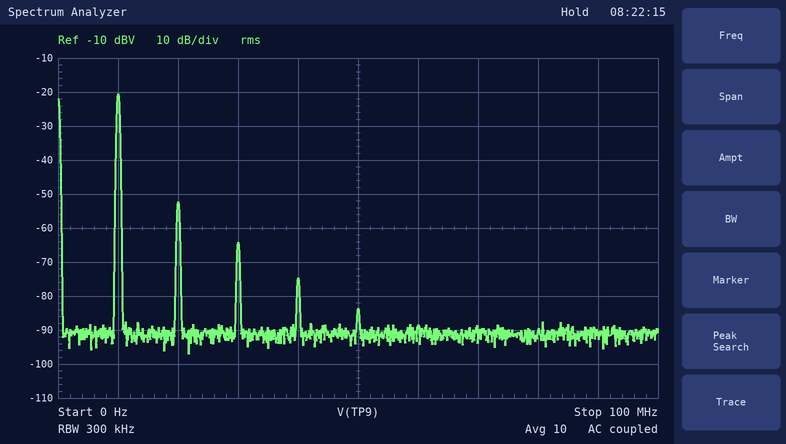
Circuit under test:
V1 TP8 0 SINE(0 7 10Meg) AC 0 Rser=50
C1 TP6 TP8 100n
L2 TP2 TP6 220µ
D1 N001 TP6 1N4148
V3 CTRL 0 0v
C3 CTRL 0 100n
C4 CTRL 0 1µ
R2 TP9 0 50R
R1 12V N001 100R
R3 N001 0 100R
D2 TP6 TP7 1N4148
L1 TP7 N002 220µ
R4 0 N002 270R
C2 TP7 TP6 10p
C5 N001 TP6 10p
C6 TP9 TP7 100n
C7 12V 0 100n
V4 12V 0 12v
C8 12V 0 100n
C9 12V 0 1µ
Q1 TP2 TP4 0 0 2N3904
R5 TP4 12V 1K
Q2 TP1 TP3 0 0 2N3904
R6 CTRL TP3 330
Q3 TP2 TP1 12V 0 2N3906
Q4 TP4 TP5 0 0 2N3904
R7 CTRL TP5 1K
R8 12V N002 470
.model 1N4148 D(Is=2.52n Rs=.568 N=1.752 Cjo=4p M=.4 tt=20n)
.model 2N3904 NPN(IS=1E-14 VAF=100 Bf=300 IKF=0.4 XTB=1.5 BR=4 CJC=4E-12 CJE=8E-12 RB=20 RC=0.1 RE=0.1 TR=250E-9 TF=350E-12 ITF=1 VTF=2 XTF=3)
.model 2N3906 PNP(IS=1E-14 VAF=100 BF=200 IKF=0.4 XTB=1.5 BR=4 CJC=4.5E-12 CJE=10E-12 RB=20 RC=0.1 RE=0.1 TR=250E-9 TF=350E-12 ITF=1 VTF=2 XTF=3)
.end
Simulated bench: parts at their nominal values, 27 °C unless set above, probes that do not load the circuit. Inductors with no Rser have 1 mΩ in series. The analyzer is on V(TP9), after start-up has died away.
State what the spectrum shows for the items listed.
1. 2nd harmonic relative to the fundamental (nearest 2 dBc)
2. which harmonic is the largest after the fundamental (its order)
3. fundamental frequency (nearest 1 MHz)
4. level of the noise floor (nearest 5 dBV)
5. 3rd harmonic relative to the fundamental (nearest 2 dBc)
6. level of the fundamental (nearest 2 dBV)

-32 dBc
2
10 MHz
-90 dBV
-44 dBc
-20 dBV
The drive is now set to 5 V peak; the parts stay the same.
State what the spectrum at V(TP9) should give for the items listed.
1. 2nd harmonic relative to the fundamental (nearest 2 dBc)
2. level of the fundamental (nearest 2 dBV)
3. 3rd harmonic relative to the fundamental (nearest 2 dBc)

-36 dBc
-24 dBV
-50 dBc
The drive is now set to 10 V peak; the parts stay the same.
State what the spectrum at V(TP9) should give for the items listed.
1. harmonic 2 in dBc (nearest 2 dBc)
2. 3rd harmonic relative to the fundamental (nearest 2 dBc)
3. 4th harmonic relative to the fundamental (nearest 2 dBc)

-20 dBc
-22 dBc
-22 dBc
